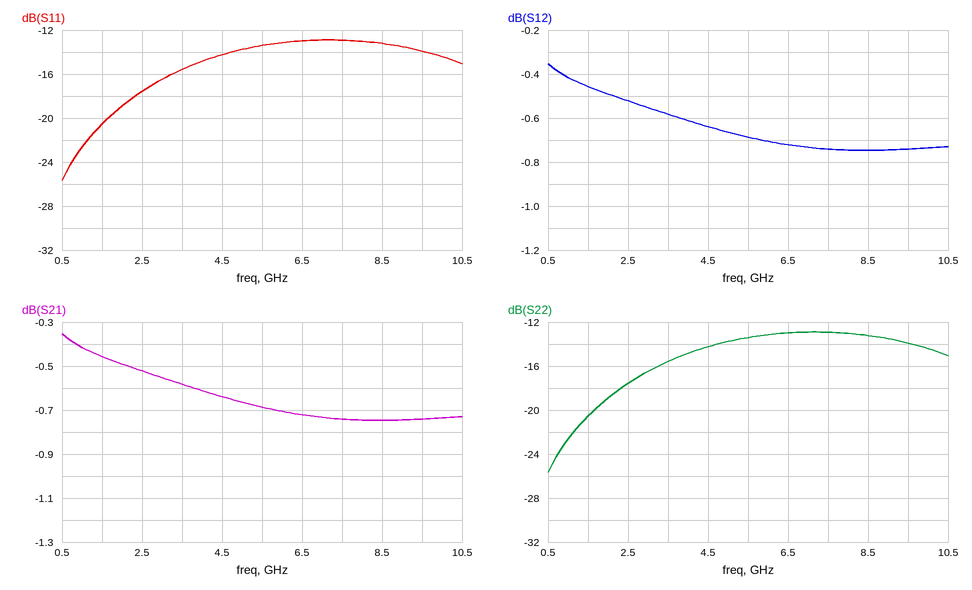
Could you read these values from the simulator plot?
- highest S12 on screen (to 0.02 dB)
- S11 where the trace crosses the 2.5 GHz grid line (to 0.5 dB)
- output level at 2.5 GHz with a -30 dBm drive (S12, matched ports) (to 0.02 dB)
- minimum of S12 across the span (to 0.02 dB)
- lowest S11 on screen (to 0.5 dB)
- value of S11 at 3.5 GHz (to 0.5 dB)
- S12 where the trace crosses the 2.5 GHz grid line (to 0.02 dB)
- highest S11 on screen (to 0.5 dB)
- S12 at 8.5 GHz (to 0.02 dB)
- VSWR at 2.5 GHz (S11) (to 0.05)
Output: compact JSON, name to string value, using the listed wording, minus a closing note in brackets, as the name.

{"highest S12 on screen": "-0.36 dB", "S11 where the trace crosses the 2.5 GHz grid line": "-17.5 dB", "output level at 2.5 GHz with a -30 dBm drive (S12, matched ports)": "-30.52 dBm", "minimum of S12 across the span": "-0.74 dB", "lowest S11 on screen": "-25.5 dB", "value of S11 at 3.5 GHz": "-15.5 dB", "S12 where the trace crosses the 2.5 GHz grid line": "-0.52 dB", "highest S11 on screen": "-13.0 dB", "S12 at 8.5 GHz": "-0.74 dB", "VSWR at 2.5 GHz (S11)": "1.30"}
